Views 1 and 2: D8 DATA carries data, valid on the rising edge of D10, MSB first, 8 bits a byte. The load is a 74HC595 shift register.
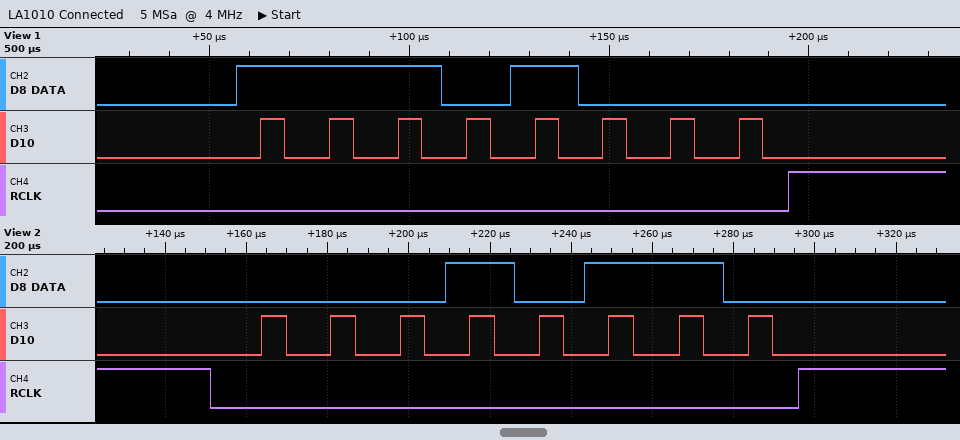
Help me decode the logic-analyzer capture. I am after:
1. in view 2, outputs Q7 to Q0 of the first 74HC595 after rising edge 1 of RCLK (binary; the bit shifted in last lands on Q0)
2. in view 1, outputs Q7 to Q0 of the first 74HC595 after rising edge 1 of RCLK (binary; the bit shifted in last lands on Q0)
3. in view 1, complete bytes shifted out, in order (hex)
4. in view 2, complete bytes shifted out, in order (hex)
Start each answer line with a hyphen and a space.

- 00010110
- 11101000
- E8
- 0x16
